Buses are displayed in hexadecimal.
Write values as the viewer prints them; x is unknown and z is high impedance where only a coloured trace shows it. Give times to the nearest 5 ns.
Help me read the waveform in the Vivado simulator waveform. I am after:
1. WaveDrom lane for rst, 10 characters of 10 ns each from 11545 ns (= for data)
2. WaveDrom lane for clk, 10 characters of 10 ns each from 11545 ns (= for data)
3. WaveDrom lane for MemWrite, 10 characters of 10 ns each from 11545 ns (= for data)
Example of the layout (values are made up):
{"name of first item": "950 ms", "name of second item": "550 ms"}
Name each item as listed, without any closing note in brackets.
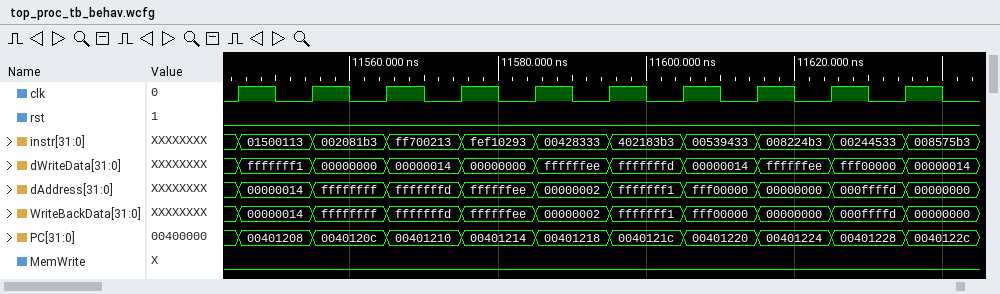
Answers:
{"WaveDrom lane for rst, 10 characters of 10 ns each from 11545 ns": "{name: 'rst', wave: '0.........'}", "WaveDrom lane for clk, 10 characters of 10 ns each from 11545 ns": "{name: 'clk', wave: 'p.........'}", "WaveDrom lane for MemWrite, 10 characters of 10 ns each from 11545 ns": "{name: 'MemWrite', wave: '0.........'}"}
